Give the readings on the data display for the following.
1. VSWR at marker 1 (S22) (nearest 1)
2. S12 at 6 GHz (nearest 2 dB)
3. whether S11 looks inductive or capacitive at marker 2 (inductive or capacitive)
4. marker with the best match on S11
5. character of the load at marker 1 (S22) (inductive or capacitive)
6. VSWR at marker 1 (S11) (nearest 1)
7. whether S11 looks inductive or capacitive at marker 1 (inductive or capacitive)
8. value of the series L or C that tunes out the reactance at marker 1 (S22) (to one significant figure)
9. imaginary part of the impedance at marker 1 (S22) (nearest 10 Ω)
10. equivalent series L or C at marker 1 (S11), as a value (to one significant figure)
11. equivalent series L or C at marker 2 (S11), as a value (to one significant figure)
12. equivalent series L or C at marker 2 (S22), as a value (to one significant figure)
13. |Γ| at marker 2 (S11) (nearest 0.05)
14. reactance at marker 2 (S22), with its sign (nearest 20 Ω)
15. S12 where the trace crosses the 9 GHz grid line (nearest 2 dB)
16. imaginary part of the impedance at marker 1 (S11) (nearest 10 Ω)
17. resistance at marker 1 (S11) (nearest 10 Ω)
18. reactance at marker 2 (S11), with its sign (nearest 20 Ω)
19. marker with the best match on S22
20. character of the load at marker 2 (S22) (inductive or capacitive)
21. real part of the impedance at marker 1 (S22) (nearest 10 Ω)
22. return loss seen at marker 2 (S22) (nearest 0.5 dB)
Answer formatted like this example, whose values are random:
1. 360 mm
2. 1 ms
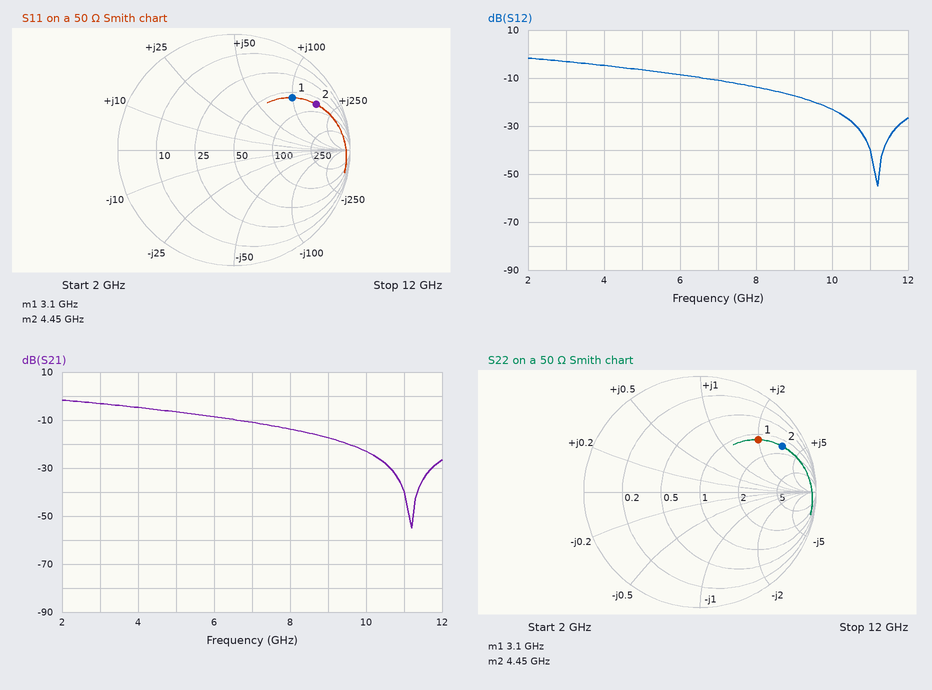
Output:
1. 5
2. -8 dB
3. inductive
4. marker 1
5. inductive
6. 5
7. inductive
8. 500 fF
9. +100 Ω
10. 5 nH
11. 6 nH
12. 6 nH
13. 0.80
14. +160 Ω
15. -18 dB
16. +100 Ω
17. 60 Ω
18. +160 Ω
19. marker 1
20. inductive
21. 60 Ω
22. 2.0 dB
